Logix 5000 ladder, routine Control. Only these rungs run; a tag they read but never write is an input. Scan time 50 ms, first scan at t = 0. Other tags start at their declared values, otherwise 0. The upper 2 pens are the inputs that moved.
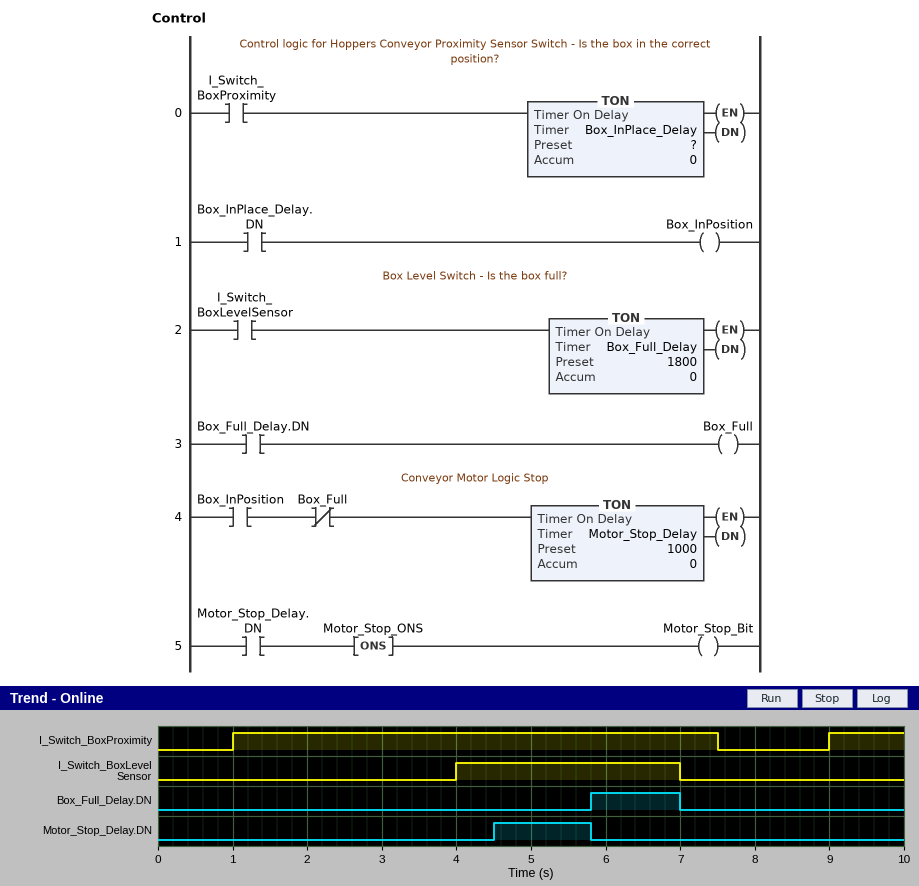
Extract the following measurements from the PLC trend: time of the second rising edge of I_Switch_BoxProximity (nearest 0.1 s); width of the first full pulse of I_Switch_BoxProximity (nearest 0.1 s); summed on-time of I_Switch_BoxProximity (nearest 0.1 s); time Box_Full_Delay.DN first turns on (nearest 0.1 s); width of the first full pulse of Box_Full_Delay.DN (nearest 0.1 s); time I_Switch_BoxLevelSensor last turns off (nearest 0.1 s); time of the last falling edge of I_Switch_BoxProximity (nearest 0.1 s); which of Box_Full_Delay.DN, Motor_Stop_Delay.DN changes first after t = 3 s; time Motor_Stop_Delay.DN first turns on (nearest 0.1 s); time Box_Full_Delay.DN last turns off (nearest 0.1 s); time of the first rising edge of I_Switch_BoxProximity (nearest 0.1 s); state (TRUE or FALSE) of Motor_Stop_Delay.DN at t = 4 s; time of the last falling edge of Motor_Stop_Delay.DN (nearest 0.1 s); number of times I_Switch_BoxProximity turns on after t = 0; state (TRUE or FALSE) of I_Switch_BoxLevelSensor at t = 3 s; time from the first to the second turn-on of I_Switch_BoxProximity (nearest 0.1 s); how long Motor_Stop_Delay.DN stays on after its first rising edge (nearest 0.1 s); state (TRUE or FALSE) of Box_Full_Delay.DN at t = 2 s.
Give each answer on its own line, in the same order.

9.0 s
6.5 s
7.5 s
5.8 s
1.2 s
7.0 s
7.5 s
Motor_Stop_Delay.DN
4.5 s
7.0 s
1.0 s
FALSE
5.8 s
2
FALSE
8.0 s
1.3 s
FALSE
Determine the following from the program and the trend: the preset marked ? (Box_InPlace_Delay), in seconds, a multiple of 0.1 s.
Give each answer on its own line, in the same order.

2.5 s
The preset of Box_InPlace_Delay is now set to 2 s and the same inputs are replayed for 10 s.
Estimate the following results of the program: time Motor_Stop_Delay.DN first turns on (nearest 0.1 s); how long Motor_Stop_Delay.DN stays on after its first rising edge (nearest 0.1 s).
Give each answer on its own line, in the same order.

4.0 s
1.8 s
